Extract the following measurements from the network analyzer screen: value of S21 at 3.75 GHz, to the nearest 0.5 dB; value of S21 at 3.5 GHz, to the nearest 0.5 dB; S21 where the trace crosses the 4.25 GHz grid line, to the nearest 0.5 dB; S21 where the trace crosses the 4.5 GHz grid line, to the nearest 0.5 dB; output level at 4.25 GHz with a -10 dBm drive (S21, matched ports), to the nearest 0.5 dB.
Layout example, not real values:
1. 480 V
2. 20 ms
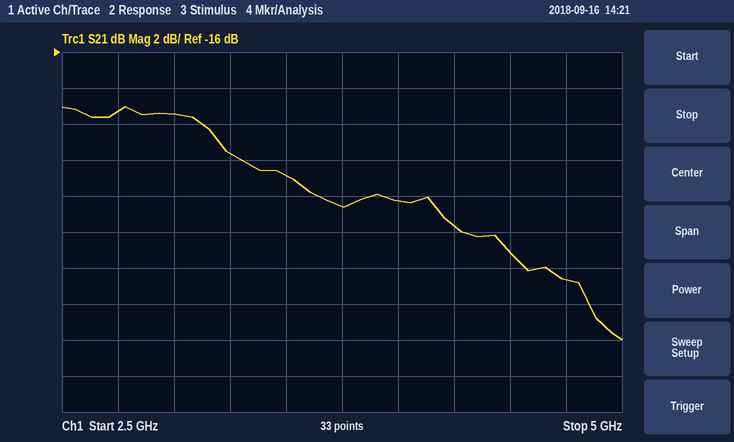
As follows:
1. -24.5 dB
2. -23.0 dB
3. -25.5 dB
4. -27.0 dB
5. -35.5 dBm
